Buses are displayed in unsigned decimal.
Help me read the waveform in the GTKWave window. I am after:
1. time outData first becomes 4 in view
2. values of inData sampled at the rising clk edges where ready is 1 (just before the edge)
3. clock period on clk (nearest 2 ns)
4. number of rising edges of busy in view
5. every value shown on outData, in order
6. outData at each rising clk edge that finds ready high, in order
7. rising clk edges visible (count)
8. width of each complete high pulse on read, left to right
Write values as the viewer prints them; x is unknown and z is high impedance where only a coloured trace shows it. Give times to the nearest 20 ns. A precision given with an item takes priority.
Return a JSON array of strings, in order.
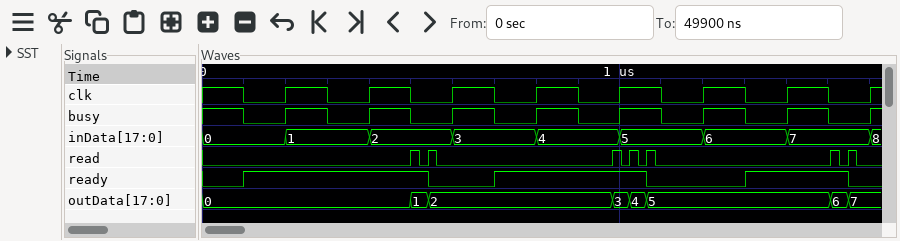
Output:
["1020 ns", "0, 1, 3, 4, 6", "200 ns", "8", "0, 1, 2, 3, 4, 5, 6, 7", "0, 0, 2, 3, 5", "8", "20 ns, 20 ns, 20 ns, 20 ns, 20 ns, 20 ns, 20 ns"]
